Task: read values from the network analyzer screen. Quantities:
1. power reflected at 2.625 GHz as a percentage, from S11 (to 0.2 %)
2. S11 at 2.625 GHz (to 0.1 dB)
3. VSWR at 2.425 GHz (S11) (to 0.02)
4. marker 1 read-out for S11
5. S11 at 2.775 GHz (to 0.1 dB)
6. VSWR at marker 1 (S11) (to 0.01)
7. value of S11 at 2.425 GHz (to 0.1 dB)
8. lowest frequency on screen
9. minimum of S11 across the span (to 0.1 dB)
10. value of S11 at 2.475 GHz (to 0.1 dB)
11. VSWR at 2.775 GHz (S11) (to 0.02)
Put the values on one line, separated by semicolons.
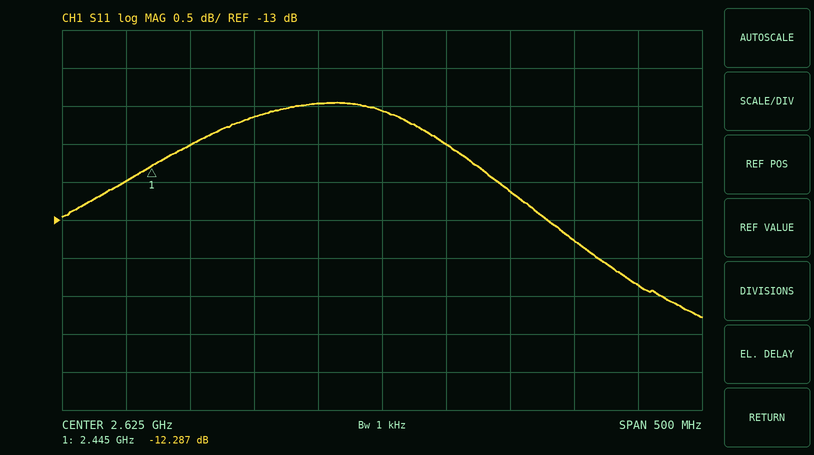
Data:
7.0 %; -11.6 dB; 1.62; -12.287 dB; -13.3 dB; 1.64; -12.5 dB; 2.375 GHz; -14.3 dB; -12.0 dB; 1.56
